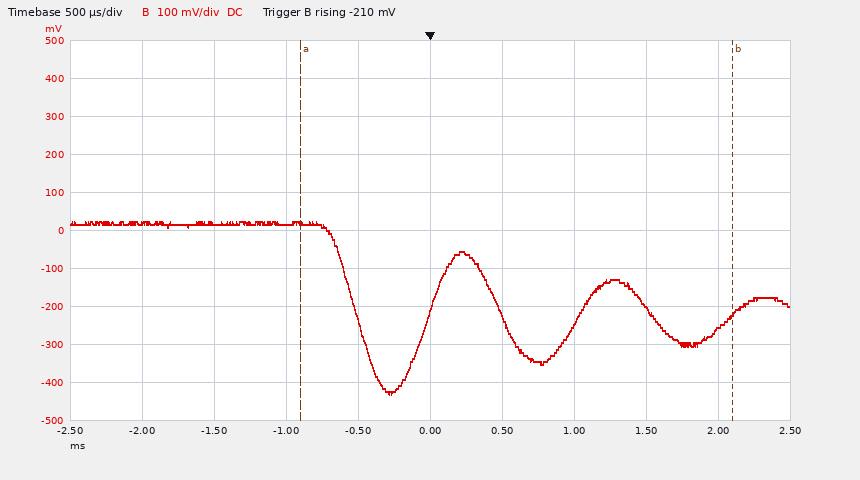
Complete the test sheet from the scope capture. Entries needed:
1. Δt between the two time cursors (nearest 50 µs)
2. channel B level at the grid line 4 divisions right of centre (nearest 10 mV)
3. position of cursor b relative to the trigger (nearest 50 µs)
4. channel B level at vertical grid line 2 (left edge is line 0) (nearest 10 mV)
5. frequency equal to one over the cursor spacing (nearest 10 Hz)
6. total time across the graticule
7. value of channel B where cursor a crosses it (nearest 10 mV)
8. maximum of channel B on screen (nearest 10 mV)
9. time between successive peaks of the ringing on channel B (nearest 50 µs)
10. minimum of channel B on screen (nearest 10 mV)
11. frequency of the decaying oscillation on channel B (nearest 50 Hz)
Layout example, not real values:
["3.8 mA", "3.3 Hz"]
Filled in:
["3.00 ms", "-260 mV", "+2.10 ms", "20 mV", "330 Hz", "5 ms", "20 mV", "20 mV", "1.05 ms", "-430 mV", "950 Hz"]
